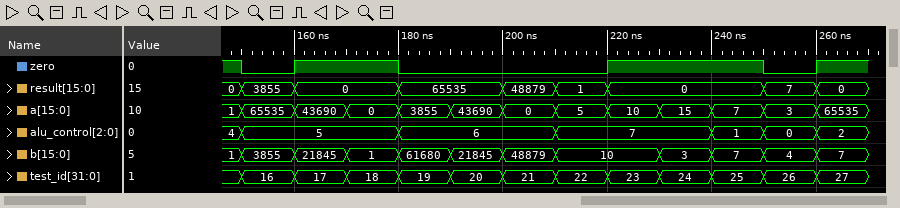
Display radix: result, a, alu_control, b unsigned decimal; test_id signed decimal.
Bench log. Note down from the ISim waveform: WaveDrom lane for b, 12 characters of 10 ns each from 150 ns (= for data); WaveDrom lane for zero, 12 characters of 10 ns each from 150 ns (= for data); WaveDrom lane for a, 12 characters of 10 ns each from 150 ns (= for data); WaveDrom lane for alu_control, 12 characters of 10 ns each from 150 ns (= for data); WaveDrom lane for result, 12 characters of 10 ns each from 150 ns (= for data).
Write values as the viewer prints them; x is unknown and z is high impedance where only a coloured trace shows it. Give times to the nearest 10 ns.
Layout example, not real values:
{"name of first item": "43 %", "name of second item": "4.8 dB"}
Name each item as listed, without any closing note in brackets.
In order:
{"WaveDrom lane for b, 12 characters of 10 ns each from 150 ns": "{name: 'b', wave: '=======.====', data: '3855 21845 1 61680 21845 48879 10 3 7 4 7'}", "WaveDrom lane for zero, 12 characters of 10 ns each from 150 ns": "{name: 'zero', wave: '01.0...1..01'}", "WaveDrom lane for a, 12 characters of 10 ns each from 150 ns": "{name: 'a', wave: '============', data: '65535 43690 0 3855 43690 0 5 10 15 7 3 65535'}", "WaveDrom lane for alu_control, 12 characters of 10 ns each from 150 ns": "{name: 'alu_control', wave: '=..=..=..===', data: '5 6 7 1 0 2'}", "WaveDrom lane for result, 12 characters of 10 ns each from 150 ns": "{name: 'result', wave: '==.=.===..==', data: '3855 0 65535 48879 1 0 7 0'}"}
